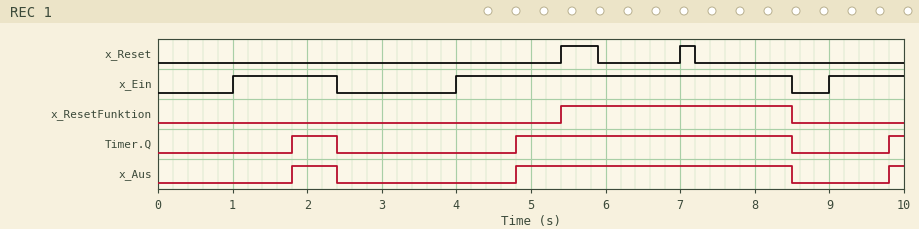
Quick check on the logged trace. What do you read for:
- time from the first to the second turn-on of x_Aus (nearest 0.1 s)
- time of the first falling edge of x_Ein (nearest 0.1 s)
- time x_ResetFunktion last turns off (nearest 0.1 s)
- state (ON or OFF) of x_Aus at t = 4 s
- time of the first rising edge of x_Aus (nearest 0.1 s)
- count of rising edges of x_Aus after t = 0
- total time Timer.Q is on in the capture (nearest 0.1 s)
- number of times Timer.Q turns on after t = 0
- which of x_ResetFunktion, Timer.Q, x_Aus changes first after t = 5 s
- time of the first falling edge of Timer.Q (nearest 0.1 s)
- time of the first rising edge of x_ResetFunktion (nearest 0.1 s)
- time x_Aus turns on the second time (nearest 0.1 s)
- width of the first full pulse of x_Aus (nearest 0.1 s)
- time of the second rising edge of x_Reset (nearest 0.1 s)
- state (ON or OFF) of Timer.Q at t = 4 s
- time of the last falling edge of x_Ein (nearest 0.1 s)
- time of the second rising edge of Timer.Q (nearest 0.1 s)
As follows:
3.0 s
2.4 s
8.5 s
OFF
1.8 s
3
4.5 s
3
x_ResetFunktion
2.4 s
5.4 s
4.8 s
0.6 s
7.0 s
OFF
8.5 s
4.8 s
